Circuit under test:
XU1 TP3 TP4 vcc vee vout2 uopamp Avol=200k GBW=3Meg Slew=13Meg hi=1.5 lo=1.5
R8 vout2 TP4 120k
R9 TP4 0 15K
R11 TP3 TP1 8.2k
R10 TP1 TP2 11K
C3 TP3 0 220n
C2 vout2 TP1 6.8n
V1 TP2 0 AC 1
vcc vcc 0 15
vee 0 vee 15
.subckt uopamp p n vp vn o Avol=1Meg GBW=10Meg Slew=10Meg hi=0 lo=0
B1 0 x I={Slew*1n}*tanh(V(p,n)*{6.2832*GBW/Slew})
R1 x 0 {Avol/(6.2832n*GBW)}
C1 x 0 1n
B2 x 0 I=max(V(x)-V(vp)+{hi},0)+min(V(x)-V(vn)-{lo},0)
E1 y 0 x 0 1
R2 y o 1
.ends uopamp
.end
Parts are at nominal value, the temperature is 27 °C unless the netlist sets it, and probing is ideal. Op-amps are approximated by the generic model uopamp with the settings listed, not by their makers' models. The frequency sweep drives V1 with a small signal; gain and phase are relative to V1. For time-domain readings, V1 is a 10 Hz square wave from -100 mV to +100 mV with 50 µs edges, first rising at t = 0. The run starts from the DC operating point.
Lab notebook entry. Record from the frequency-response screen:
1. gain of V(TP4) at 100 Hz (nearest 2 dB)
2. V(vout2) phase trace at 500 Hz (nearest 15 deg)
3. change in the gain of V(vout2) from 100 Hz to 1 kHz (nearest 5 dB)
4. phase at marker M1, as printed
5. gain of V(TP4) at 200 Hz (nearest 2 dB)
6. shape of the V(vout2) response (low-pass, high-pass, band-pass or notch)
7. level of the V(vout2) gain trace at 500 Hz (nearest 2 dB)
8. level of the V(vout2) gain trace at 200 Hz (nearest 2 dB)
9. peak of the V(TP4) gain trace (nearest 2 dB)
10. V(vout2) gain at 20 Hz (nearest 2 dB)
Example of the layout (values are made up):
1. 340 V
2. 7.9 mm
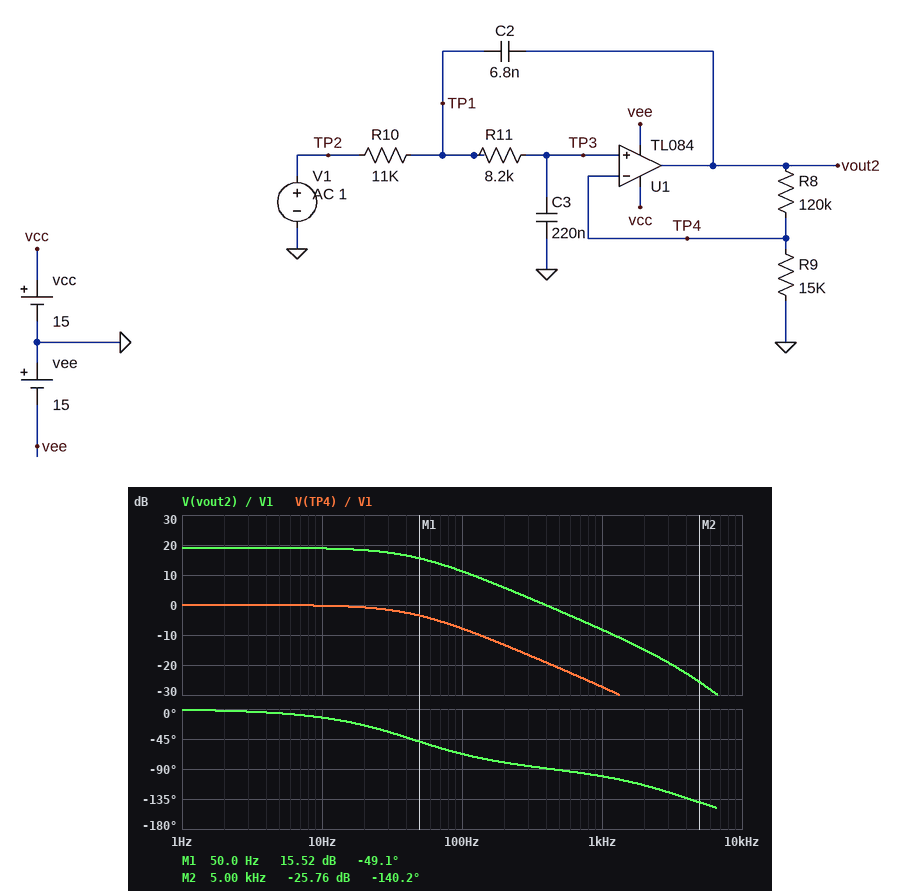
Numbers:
1. -8 dB
2. -90 deg
3. -20 dB
4. -49.1 deg
5. -14 dB
6. low-pass
7. -2 dB
8. 6 dB
9. 0 dB
10. 18 dB
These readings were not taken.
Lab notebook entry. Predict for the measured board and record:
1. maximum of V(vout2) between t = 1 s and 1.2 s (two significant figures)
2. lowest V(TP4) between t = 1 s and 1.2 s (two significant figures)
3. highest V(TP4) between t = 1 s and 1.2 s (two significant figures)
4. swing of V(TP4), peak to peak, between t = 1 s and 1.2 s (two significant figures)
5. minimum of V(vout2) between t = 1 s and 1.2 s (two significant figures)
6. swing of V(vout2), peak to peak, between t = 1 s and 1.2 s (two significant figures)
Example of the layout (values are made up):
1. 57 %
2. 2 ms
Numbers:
1. 900 mV
2. -100 mV
3. 100 mV
4. 200 mV
5. -900 mV
6. 1.8 V
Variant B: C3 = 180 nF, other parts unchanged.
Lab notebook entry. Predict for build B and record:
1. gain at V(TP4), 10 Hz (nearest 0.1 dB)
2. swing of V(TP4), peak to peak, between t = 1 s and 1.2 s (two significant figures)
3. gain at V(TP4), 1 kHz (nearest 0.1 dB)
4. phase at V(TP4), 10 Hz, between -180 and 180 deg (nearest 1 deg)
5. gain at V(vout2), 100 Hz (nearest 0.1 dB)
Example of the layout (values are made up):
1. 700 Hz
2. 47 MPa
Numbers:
1. -0.1 dB
2. 200 mV
3. -25.2 dB
4. -10 deg
5. 12.9 dB
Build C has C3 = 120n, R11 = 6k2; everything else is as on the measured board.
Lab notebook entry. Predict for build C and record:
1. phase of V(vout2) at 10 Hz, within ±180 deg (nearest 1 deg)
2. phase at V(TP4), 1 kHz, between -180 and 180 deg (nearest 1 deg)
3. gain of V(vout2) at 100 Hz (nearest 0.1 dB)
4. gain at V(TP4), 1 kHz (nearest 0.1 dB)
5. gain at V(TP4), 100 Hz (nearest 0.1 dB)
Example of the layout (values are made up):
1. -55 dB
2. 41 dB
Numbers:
1. -5 deg
2. -98 deg
3. 16.5 dB
4. -19.4 dB
5. -2.6 dB
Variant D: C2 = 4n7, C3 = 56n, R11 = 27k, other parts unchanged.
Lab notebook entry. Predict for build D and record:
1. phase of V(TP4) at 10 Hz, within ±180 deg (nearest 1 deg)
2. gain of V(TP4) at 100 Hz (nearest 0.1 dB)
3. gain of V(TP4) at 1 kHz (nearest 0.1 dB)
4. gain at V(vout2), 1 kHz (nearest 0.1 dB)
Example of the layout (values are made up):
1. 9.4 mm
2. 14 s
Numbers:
1. -6 deg
2. -3.2 dB
3. -20.8 dB
4. -1.7 dB
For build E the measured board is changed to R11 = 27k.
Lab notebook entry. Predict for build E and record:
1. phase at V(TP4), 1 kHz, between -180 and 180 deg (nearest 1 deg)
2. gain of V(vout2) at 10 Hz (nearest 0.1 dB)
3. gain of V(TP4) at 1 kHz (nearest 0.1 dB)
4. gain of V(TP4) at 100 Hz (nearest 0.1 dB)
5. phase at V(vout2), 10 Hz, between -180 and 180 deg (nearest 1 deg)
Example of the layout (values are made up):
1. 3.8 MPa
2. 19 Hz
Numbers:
1. -109 deg
2. 18.2 dB
3. -34.2 dB
4. -13.9 dB
5. -26 deg
